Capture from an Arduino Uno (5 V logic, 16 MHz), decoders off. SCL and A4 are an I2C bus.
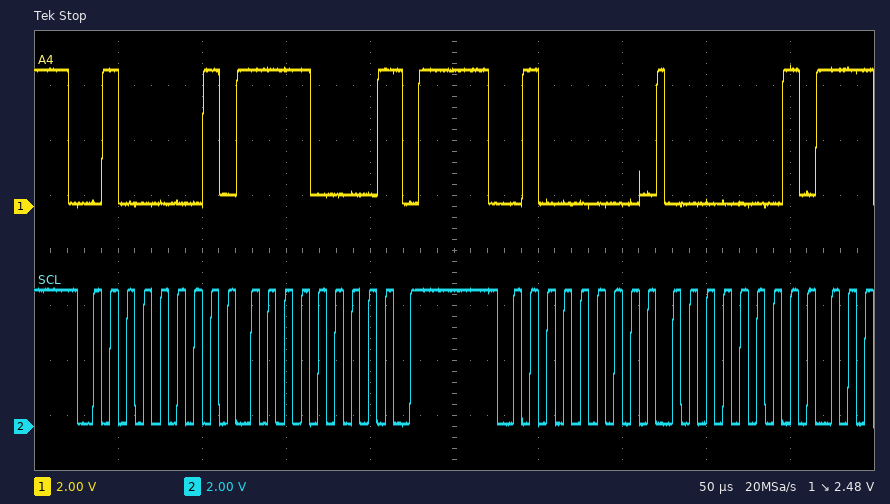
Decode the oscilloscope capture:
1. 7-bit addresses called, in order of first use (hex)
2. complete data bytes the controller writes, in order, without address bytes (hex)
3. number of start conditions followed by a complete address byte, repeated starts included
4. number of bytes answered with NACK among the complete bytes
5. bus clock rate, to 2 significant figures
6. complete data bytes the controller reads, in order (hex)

0x20
01
2
1
100 kHz
F0
